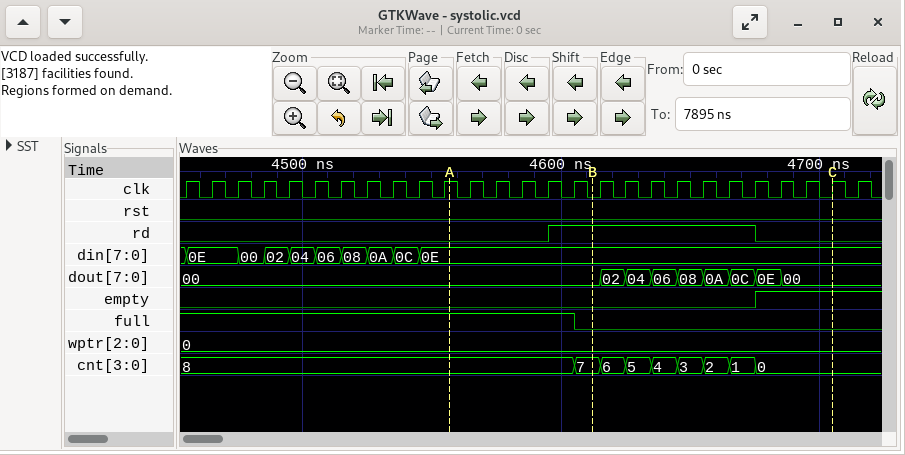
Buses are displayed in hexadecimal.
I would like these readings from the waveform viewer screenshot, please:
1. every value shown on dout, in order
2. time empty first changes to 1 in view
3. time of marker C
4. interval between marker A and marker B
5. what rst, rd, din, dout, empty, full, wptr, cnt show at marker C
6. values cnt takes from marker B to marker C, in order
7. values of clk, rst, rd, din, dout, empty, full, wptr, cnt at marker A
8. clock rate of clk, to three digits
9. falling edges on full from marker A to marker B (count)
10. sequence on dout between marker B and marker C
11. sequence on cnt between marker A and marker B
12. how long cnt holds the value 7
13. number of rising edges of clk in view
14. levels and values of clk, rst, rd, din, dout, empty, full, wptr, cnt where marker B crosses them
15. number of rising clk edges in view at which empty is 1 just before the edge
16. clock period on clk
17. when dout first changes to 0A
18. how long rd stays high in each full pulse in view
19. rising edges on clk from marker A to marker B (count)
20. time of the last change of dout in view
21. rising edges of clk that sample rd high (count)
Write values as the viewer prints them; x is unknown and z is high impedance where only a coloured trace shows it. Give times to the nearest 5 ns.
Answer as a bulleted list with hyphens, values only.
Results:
- 00, 02, 04, 06, 08, 0A, 0C, 0E, 00
- 4675 ns
- 4705 ns
- 55 ns
- rst=0, rd=0, din=0E, dout=00, empty=1, full=0, wptr=0, cnt=0
- 7, 6, 5, 4, 3, 2, 1, 0
- clk=1, rst=0, rd=0, din=0E, dout=00, empty=0, full=1, wptr=0, cnt=8
- 100 MHz
- 1
- 00, 02, 04, 06, 08, 0A, 0C, 0E, 00
- 8, 7
- 10 ns
- 27
- clk=0, rst=0, rd=1, din=0E, dout=00, empty=0, full=0, wptr=0, cnt=7
- 4
- 10 ns
- 4655 ns
- 80 ns
- 5
- 4685 ns
- 8
